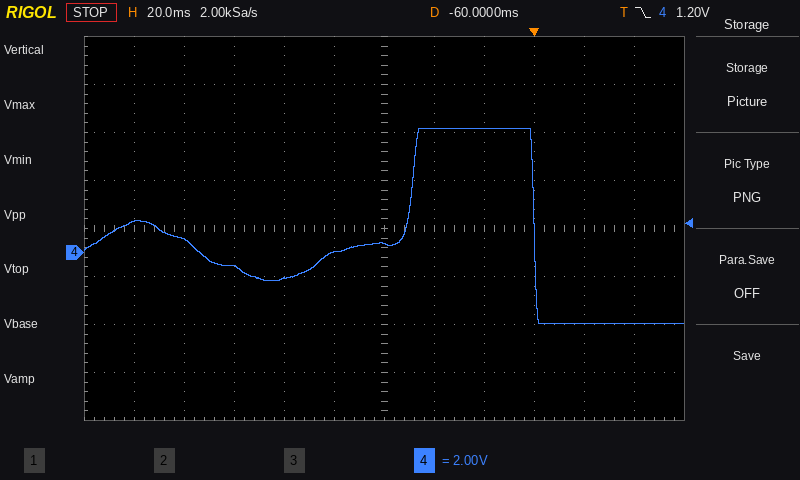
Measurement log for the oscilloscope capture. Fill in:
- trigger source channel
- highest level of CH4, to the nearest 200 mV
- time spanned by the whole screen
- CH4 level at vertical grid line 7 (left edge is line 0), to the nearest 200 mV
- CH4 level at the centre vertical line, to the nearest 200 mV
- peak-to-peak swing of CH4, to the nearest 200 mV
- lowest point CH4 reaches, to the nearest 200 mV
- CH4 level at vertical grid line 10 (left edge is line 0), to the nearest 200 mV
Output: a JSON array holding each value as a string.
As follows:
["CH4", "5.2 V", "240 ms", "5.2 V", "400 mV", "8.2 V", "-3.0 V", "-3.0 V"]
